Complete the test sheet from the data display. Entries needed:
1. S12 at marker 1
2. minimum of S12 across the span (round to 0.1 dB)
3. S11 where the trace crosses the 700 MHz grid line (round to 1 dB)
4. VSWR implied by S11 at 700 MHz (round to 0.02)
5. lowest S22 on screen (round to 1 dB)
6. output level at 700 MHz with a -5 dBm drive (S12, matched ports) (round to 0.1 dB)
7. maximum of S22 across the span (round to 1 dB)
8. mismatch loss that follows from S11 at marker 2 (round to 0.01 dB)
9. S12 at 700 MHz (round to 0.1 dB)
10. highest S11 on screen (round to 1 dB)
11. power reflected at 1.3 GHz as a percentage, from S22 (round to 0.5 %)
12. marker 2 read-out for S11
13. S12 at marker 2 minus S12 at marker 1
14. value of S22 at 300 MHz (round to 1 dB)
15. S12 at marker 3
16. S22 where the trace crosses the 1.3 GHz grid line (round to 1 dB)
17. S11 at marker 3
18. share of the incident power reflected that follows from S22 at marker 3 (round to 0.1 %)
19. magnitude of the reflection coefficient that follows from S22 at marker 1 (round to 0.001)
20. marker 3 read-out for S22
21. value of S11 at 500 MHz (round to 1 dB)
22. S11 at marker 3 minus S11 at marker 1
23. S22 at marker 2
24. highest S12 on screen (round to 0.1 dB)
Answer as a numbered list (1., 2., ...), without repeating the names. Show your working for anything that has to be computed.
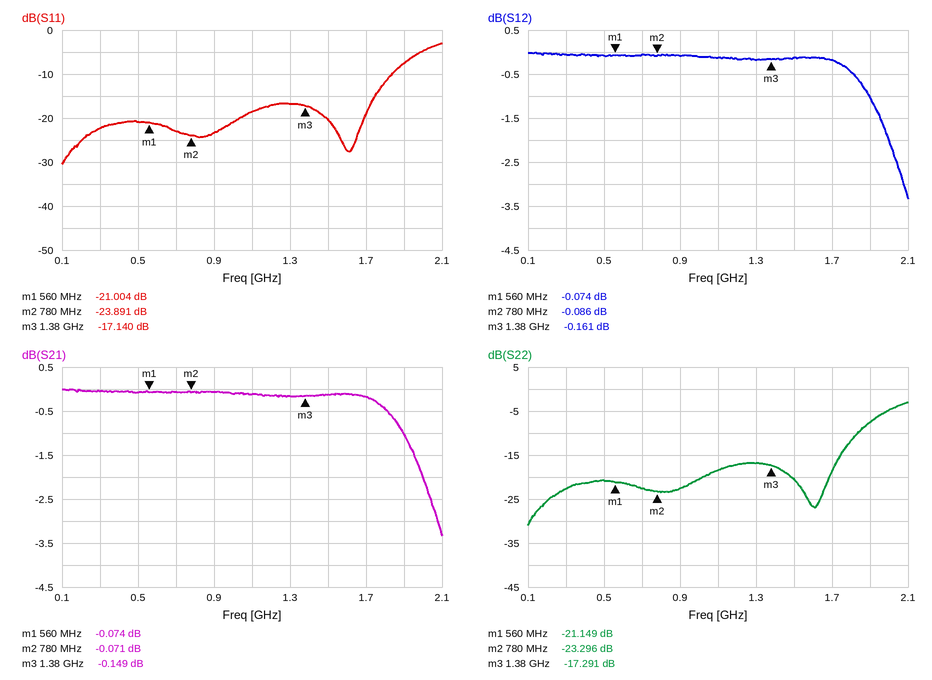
1. -0.074 dB
2. -3.3 dB
3. -23 dB
4. |Γ| = 10^(-23/20) = 0.0708; VSWR = (1 + 0.0708)/(1 − 0.0708) ≈ 1.15, so 1.16 to the nearest 0.02
5. -31 dB
6. -5 dBm + (-0.1 dB) = -5.1 dBm
7. -3 dB
8. −10 log10(1 − 10^(-23.891/10)) ≈ 0.02 dB
9. -0.1 dB
10. -3 dB
11. 10^(-17/10) ≈ 2.0 %
12. -23.891 dB
13. -0.086 − (-0.074) = -0.012 dB
14. -23 dB
15. -0.161 dB
16. -17 dB
17. -17.140 dB
18. 10^(-17.291/10) ≈ 1.9 %
19. 10^(-21.149/20) ≈ 0.088
20. -17.291 dB
21. -21 dB
22. -17.14 − (-21.004) = 3.864 dB
23. -23.296 dB
24. 0.0 dB
